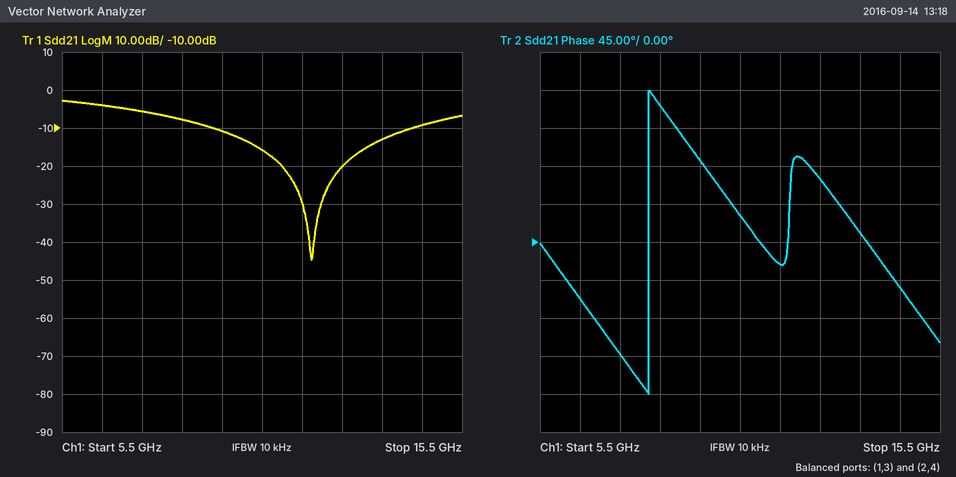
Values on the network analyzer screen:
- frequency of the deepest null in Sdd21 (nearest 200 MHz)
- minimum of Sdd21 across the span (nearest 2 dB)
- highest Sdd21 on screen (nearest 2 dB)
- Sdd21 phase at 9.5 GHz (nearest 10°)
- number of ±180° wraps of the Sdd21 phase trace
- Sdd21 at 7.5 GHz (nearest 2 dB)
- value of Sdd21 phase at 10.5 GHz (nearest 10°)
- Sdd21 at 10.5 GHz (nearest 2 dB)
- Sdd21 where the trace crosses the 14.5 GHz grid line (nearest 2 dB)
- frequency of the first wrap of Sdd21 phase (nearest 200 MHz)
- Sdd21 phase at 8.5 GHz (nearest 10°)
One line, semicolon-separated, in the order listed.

11.8 GHz; -44 dB; -2 dB; 100°; 1; -6 dB; 30°; -16 dB; -10 dB; 8.2 GHz; 160°
